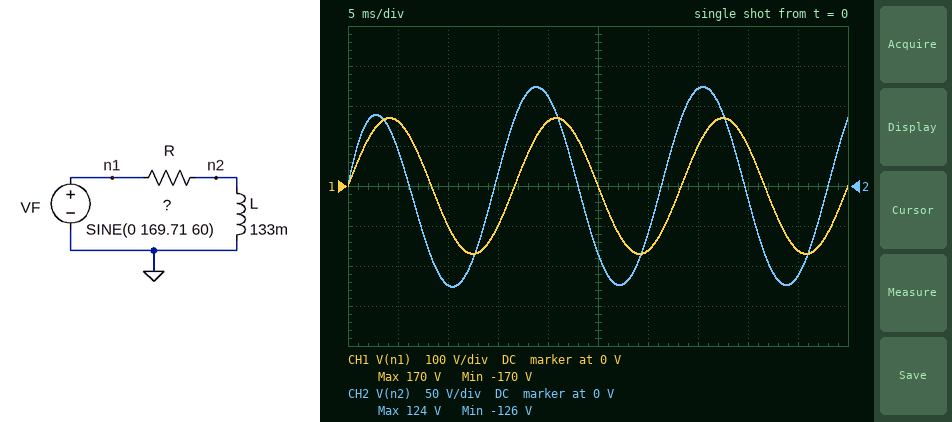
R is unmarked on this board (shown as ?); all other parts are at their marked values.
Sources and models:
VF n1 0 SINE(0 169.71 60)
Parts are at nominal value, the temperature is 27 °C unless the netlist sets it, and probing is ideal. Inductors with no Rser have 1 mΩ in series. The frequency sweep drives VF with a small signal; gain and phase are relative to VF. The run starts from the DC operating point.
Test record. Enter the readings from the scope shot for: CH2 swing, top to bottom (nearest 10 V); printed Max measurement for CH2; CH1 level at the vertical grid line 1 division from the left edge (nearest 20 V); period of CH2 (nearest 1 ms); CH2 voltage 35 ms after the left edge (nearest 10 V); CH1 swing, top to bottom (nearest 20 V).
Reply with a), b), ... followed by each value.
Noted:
a) 250 V
b) 124 V
c) 160 V
d) 17 ms
e) 120 V
f) 340 V
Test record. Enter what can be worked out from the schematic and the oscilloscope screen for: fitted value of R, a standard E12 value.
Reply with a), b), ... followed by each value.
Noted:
a) 47 Ω
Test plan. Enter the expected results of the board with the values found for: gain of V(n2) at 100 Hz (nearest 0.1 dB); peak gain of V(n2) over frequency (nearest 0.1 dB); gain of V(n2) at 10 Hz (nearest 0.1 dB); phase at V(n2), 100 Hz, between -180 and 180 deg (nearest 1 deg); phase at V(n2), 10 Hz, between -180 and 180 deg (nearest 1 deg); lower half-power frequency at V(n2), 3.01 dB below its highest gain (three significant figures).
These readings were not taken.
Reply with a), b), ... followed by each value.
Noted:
a) -1.2 dB
b) 0 dB
c) -15.1 dB
d) 29 deg
e) 80 deg
f) 56.2 Hz
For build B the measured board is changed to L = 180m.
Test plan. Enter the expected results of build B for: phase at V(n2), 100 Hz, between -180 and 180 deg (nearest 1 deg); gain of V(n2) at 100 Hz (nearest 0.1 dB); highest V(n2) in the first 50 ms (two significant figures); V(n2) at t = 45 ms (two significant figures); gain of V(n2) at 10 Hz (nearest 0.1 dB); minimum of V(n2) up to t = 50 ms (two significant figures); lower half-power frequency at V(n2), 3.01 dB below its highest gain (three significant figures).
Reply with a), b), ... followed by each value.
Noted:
a) 23 deg
b) -0.7 dB
c) 140 V
d) -130 V
e) -12.6 dB
f) -140 V
g) 41.6 Hz
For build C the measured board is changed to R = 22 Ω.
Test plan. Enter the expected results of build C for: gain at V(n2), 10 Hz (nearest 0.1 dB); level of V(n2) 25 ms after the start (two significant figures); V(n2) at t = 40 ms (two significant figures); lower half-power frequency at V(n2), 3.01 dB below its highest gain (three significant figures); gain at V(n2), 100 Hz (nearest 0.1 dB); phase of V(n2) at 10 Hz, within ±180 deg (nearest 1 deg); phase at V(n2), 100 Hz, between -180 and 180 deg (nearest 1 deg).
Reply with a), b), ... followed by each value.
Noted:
a) -9.0 dB
b) -63 V
c) 33 V
d) 26.3 Hz
e) -0.3 dB
f) 69 deg
g) 15 deg
